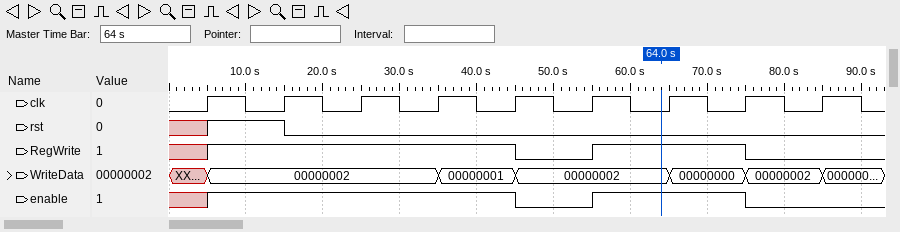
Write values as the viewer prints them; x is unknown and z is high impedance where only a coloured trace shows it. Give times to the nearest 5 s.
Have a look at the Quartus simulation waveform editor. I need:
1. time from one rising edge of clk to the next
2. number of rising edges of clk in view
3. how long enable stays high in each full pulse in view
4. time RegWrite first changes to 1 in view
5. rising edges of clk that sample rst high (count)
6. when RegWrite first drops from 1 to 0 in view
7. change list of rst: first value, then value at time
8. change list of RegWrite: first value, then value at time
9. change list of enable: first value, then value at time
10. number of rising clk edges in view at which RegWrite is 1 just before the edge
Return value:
10 s
9
20 s
5 s
1
45 s
x, 1 at 5 s, 0 at 15 s
x, 1 at 5 s, 0 at 45 s, 1 at 55 s, 0 at 75 s
x, 1 at 5 s, 0 at 45 s, 1 at 55 s, 0 at 75 s
6
